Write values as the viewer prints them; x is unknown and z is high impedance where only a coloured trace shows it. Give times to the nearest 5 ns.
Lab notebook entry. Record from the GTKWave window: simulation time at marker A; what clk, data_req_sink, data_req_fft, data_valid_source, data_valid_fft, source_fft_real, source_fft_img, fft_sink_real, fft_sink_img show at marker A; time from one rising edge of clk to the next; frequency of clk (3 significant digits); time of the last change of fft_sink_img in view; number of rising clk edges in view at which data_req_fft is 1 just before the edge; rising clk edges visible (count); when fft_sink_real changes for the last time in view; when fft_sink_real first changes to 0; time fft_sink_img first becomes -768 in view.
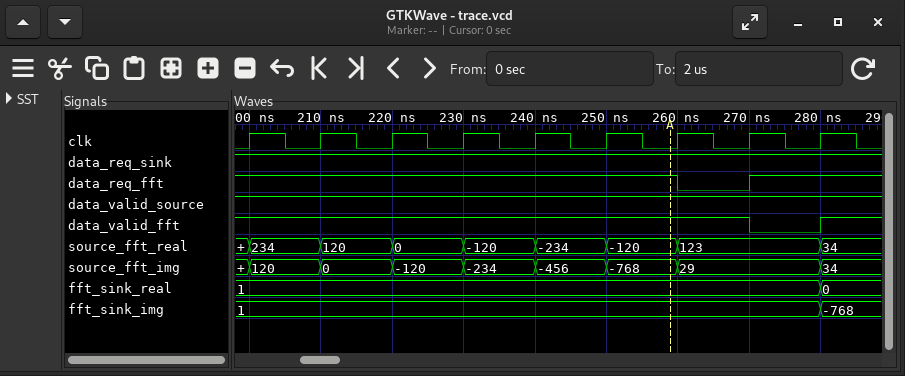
260 ns
clk=0, data_req_sink=1, data_req_fft=1, data_valid_source=1, data_valid_fft=1, source_fft_real=-120, source_fft_img=-768, fft_sink_real=1, fft_sink_img=1
10 ns
100 MHz
280 ns
8
9
280 ns
280 ns
280 ns
